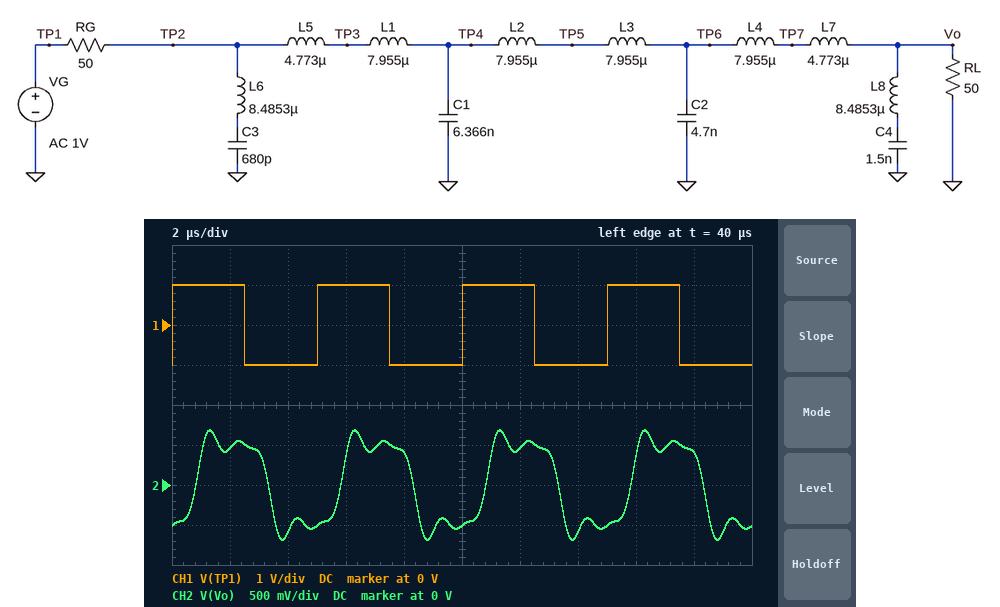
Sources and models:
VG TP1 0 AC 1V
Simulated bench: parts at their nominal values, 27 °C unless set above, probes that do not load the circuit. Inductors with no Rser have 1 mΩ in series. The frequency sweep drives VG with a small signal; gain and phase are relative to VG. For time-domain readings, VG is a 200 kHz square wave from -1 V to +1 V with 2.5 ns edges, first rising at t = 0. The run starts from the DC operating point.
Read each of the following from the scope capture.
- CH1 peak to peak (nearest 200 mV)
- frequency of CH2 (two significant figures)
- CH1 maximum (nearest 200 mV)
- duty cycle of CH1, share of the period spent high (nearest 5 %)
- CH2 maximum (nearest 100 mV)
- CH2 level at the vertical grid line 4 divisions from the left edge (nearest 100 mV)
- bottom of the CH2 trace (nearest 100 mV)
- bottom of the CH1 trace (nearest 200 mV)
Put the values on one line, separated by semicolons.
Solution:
2.0 V; 200 kHz; 1.0 V; 50 %; 700 mV; 400 mV; -700 mV; -1.0 V
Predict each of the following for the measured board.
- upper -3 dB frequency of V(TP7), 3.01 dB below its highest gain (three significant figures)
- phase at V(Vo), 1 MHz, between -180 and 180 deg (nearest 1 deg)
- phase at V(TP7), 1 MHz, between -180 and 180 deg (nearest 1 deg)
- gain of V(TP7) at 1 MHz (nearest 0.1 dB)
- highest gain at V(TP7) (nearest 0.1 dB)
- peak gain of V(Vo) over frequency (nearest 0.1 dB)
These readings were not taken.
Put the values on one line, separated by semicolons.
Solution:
866 kHz; 19 deg; 73 deg; -10.9 dB; -6.0 dB; -6.0 dB
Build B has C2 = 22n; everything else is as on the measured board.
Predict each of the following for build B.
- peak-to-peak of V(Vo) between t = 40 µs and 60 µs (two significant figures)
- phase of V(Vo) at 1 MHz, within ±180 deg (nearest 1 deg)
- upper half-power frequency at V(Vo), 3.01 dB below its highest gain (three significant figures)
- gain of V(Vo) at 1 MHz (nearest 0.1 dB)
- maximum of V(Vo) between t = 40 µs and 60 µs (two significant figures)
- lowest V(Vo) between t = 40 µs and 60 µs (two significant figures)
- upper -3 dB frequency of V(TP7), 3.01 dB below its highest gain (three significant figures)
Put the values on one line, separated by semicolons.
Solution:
1.0 V; -65 deg; 338 kHz; -30.3 dB; 510 mV; -510 mV; 331 kHz
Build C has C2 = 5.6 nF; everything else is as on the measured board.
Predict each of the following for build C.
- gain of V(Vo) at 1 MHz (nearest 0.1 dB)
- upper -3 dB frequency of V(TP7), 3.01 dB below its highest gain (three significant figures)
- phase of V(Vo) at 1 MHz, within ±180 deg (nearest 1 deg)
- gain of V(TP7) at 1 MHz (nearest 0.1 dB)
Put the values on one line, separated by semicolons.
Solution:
-10.0 dB; 910 kHz; -14 deg; -12.6 dB
